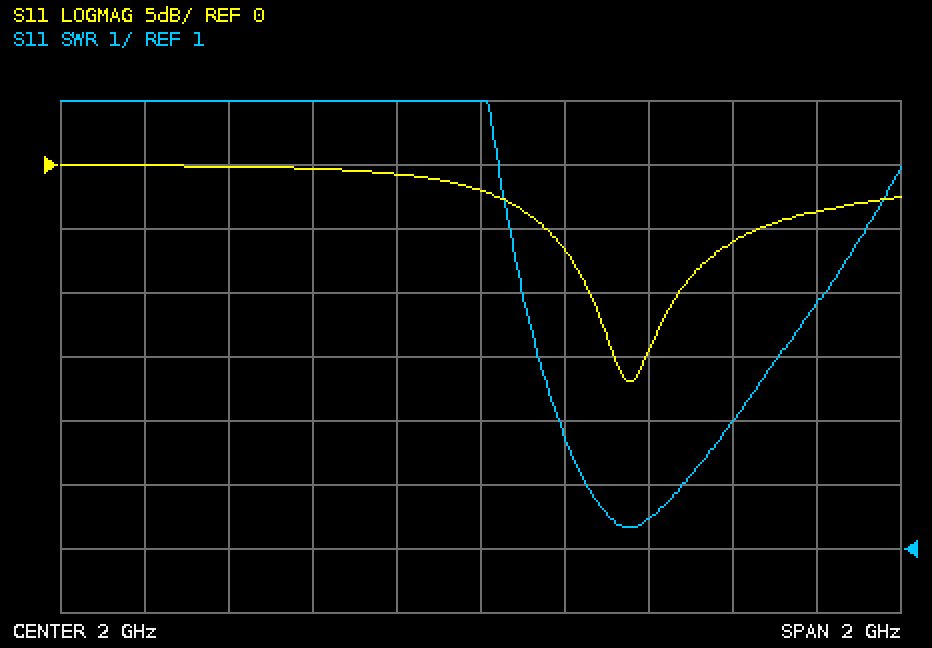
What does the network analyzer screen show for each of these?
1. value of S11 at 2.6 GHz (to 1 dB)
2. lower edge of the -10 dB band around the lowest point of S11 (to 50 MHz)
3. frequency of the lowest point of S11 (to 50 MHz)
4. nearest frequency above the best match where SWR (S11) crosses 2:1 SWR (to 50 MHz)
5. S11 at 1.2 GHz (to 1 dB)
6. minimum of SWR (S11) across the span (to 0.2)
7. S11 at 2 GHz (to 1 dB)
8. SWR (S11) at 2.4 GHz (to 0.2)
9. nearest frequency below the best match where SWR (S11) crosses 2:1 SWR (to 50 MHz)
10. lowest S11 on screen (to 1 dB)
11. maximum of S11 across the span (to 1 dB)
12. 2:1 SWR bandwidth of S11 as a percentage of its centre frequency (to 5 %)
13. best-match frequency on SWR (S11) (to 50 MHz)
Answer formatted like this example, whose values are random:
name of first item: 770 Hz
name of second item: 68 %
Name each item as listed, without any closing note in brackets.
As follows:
value of S11 at 2.6 GHz: -6 dB
lower edge of the -10 dB band around the lowest point of S11: 2.25 GHz
frequency of the lowest point of S11: 2.35 GHz
nearest frequency above the best match where SWR (S11) crosses 2:1 SWR: 2.50 GHz
S11 at 1.2 GHz: 0 dB
minimum of SWR (S11) across the span: 1.4
S11 at 2 GHz: -2 dB
SWR (S11) at 2.4 GHz: 1.4
nearest frequency below the best match where SWR (S11) crosses 2:1 SWR: 2.25 GHz
lowest S11 on screen: -17 dB
maximum of S11 across the span: 0 dB
2:1 SWR bandwidth of S11 as a percentage of its centre frequency: 10 %
best-match frequency on SWR (S11): 2.35 GHz
